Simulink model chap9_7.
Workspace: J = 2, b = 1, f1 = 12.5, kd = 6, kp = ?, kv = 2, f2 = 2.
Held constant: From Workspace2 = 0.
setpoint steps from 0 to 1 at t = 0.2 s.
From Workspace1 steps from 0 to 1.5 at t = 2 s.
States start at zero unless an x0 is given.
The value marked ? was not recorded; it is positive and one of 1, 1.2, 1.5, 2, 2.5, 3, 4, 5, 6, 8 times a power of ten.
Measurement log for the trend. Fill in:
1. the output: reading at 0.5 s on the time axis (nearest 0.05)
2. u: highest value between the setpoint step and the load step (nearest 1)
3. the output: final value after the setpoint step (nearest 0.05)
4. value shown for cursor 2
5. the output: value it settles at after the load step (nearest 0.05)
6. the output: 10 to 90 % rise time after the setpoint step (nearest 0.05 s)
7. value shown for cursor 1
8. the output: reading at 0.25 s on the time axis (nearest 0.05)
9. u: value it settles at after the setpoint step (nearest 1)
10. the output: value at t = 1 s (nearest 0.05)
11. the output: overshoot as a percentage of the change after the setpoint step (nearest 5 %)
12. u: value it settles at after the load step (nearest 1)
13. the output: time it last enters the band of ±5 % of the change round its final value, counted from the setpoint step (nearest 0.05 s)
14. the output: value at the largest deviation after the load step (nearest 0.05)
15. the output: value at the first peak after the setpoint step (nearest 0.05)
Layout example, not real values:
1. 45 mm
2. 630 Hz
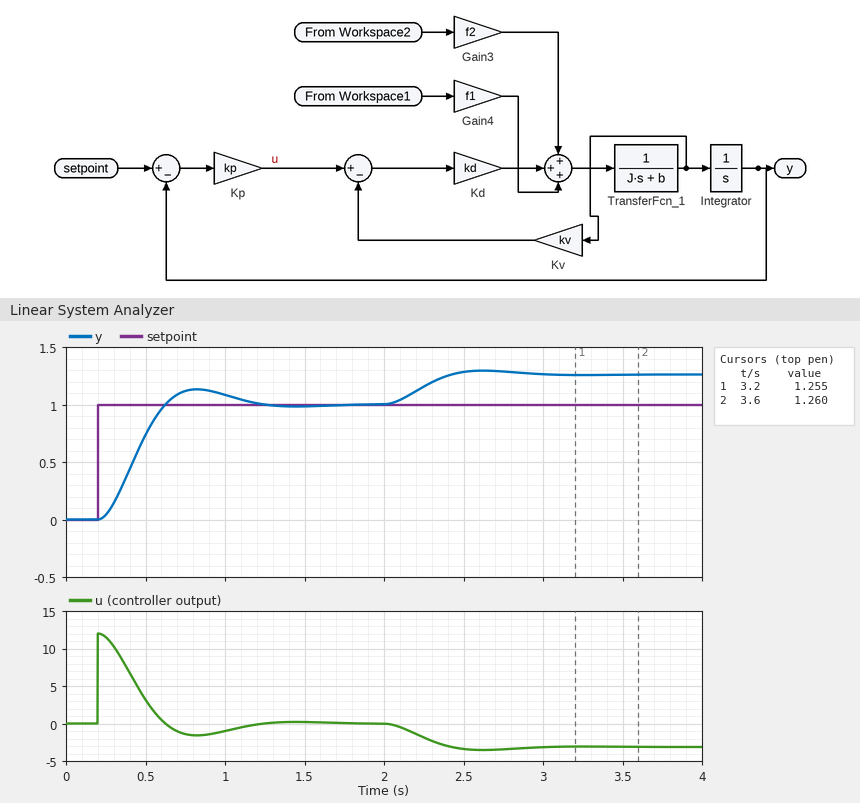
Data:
1. 0.75
2. 12
3. 1.00
4. 1.260
5. 1.25
6. 0.30 s
7. 1.255
8. 0.05
9. 0
10. 1.10
11. 15 %
12. -3
13. 0.90 s
14. 1.30
15. 1.15
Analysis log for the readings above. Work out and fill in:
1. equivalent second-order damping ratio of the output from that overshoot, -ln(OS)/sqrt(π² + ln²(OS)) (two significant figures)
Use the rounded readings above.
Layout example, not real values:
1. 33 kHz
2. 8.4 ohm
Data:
1. 0.52
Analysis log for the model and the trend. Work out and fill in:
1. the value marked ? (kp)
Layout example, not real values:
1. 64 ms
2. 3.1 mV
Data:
1. 12
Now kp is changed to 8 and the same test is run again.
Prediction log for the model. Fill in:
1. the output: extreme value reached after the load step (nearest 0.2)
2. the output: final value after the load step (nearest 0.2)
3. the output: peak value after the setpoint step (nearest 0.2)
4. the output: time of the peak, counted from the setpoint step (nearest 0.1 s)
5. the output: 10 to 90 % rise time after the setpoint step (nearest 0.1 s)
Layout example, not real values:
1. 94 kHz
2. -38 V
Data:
1. 1.4
2. 1.4
3. 1.0
4. 0.9 s
5. 0.4 s
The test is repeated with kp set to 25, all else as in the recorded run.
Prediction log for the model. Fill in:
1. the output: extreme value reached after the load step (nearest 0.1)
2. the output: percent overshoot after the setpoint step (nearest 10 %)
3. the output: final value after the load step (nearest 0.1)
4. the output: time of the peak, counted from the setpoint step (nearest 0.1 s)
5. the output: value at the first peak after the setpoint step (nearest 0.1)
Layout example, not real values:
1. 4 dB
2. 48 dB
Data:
1. 1.2
2. 30 %
3. 1.1
4. 0.4 s
5. 1.3
